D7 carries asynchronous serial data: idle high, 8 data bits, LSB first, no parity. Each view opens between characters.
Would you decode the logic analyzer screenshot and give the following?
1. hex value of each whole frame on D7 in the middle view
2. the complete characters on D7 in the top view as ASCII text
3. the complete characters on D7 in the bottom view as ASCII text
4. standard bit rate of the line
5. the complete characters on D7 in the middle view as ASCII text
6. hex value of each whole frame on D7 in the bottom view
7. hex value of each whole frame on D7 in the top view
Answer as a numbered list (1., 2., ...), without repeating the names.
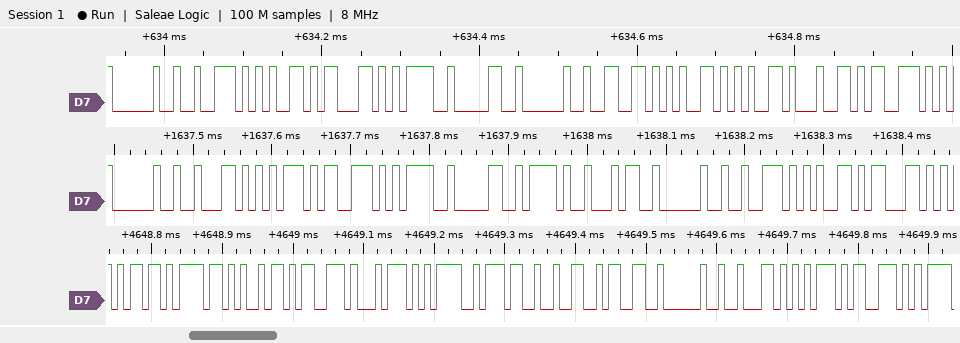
1. 20, 62, 75, 73, 3D, 30, 2F, 34, 20, 72, 65, 63
2. " rec=0 feeds"
3. "moist=723 bus"
4. 115200 baud
5. " bus=0/4 rec"
6. 6D, 6F, 69, 73, 74, 3D, 37, 32, 33, 20, 62, 75, 73
7. 20, 72, 65, 63, 3D, 30, 20, 66, 65, 65, 64, 73
